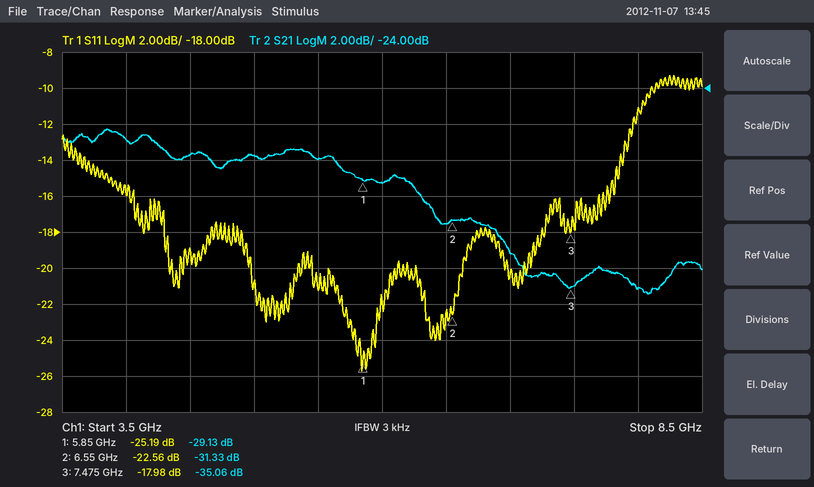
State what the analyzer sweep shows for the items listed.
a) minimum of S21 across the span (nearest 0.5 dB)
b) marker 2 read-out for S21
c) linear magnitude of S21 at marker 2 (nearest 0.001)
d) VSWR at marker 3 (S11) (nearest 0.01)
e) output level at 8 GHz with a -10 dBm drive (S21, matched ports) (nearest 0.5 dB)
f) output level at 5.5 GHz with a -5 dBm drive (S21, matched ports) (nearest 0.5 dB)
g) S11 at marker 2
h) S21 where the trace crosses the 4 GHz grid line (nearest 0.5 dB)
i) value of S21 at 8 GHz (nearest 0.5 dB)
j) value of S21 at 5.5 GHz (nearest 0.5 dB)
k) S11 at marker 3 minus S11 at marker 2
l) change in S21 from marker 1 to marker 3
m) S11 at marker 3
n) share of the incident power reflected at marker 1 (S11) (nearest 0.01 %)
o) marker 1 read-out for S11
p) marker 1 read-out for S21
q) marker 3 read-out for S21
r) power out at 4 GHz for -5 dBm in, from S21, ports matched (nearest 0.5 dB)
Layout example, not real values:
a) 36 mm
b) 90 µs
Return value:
a) -35.5 dB
b) -31.33 dB
c) 0.027
d) 1.29
e) -45.0 dBm
f) -33.0 dBm
g) -22.56 dB
h) -27.0 dB
i) -35.0 dB
j) -28.0 dB
k) 4.58 dB
l) -5.93 dB
m) -17.98 dB
n) 0.30 %
o) -25.19 dB
p) -29.13 dB
q) -35.06 dB
r) -32.0 dBm
